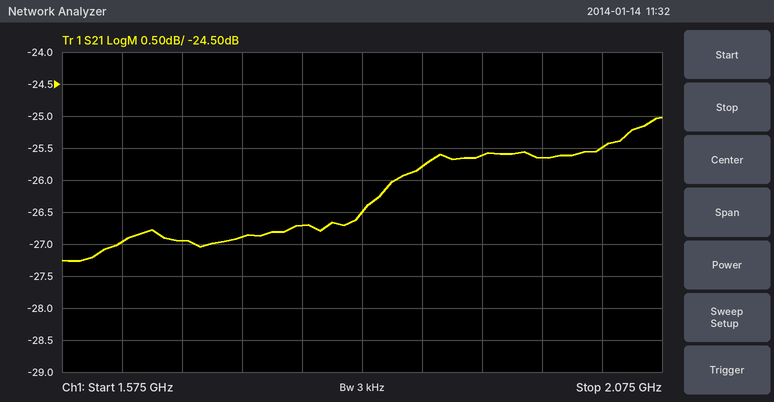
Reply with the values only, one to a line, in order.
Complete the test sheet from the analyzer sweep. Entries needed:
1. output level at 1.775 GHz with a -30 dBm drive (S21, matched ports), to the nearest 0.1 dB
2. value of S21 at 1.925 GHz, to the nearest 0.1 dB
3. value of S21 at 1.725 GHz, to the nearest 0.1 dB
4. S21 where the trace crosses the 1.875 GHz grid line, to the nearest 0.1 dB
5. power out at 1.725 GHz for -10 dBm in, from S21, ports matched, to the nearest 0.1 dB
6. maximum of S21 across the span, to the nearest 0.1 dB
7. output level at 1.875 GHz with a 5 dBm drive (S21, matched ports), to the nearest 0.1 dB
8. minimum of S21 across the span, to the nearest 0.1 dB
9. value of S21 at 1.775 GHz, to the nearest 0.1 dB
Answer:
-56.7 dBm
-25.6 dB
-26.9 dB
-25.8 dB
-36.9 dBm
-25.0 dB
-20.8 dBm
-27.3 dB
-26.7 dB
